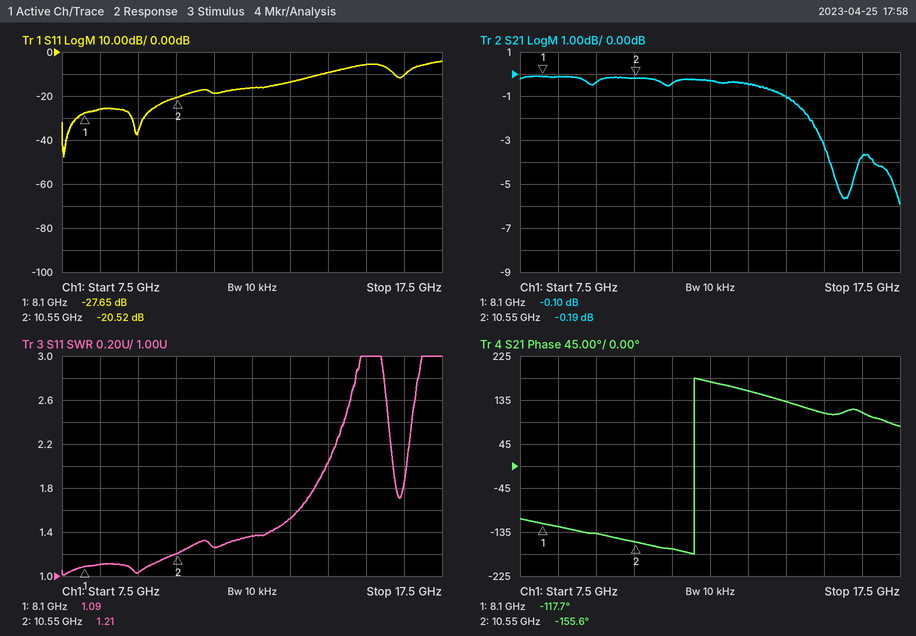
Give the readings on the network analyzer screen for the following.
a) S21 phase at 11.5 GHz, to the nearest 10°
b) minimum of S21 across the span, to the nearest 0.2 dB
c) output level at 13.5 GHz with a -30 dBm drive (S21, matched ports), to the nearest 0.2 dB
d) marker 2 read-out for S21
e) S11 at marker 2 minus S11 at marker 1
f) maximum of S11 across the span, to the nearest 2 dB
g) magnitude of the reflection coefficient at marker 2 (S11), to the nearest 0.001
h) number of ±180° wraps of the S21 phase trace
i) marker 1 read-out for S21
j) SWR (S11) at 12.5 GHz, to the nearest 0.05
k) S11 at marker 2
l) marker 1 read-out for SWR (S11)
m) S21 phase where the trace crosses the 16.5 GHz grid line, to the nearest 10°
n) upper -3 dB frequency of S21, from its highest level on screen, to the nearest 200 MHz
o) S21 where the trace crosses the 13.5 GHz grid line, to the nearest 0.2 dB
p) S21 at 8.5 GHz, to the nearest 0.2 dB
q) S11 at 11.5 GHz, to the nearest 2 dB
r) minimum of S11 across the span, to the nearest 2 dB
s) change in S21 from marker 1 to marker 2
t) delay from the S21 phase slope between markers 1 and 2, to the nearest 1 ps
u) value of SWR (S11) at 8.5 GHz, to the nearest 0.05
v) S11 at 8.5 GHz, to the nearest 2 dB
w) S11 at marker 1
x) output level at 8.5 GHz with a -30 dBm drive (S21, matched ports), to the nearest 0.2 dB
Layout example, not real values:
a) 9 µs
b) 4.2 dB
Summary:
a) -170°
b) -6.0 dB
c) -30.4 dBm
d) -0.19 dB
e) 7.13 dB
f) -4 dB
g) 0.094
h) 1
i) -0.10 dB
j) 1.35
k) -20.52 dB
l) 1.09
m) 110°
n) 15.4 GHz
o) -0.4 dB
p) -0.2 dB
q) -18 dB
r) -48 dB
s) -0.09 dB
t) 43 ps
u) 1.10
v) -26 dB
w) -27.65 dB
x) -30.2 dBm
